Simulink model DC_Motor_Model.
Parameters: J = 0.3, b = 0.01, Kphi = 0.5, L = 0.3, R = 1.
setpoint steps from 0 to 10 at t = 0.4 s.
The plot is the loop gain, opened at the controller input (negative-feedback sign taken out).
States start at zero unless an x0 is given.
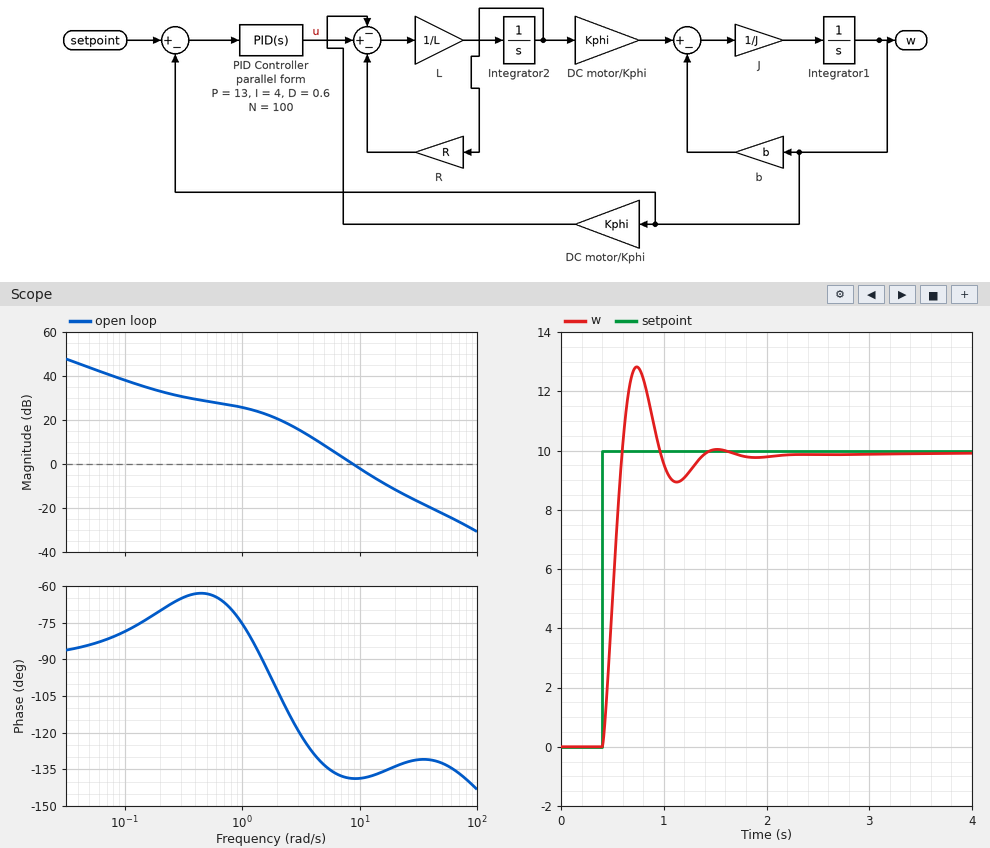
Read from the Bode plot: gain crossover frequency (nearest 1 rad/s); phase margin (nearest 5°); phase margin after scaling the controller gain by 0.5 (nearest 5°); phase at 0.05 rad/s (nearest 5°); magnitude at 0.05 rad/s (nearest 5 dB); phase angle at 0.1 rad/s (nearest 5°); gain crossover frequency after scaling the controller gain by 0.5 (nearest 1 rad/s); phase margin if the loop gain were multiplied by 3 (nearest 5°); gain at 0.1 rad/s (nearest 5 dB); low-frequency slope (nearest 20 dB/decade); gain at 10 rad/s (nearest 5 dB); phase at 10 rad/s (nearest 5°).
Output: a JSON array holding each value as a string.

["9 rad/s", "40°", "45°", "-85°", "45 dB", "-80°", "6 rad/s", "45°", "40 dB", "-20 dB/decade", "0 dB", "-140°"]
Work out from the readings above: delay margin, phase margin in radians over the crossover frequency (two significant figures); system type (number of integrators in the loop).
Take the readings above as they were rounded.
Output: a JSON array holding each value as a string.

["0.078 s", "1"]
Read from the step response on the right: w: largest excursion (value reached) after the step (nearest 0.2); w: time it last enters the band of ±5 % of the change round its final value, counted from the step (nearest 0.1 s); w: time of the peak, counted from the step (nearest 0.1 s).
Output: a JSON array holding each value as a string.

["12.8", "0.9 s", "0.3 s"]
